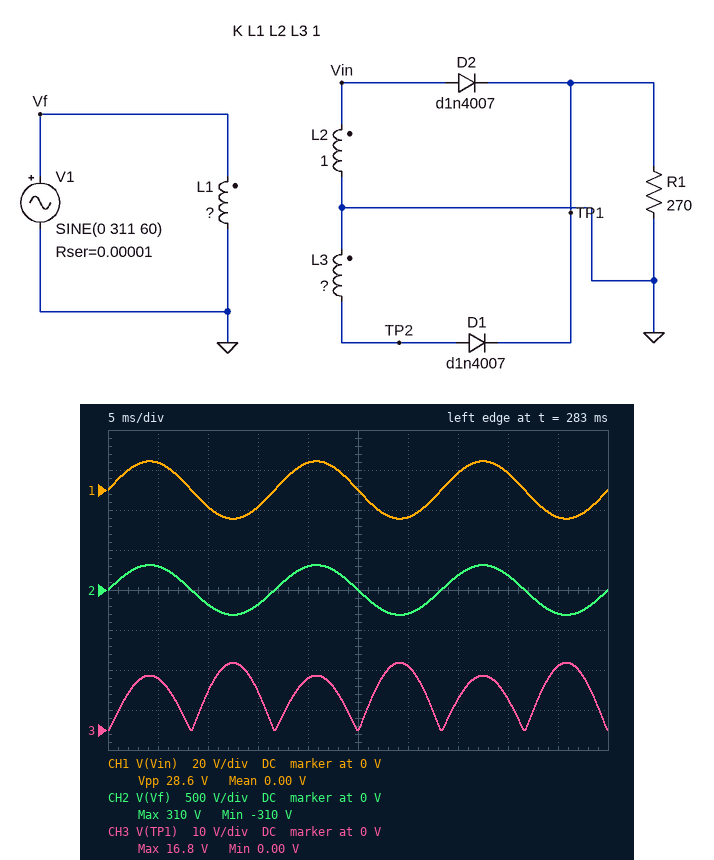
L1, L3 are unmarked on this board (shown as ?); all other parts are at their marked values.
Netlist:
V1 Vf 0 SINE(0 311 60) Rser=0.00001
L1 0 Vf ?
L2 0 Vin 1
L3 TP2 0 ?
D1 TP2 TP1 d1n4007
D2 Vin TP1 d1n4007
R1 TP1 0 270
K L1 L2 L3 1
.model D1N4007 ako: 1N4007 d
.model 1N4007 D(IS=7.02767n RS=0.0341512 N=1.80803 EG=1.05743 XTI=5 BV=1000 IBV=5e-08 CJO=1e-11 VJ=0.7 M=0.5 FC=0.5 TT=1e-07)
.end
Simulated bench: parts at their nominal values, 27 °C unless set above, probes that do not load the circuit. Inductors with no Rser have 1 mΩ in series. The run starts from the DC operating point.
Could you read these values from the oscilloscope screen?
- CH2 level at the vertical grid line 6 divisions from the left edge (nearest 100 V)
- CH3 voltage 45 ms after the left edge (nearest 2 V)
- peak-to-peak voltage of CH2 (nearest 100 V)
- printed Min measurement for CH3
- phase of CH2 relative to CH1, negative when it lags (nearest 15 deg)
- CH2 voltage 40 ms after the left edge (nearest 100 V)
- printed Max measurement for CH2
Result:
-300 V
16 V
600 V
0.00 V
0 deg
200 V
310 V
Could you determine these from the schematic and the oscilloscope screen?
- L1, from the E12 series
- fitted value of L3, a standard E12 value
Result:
470 H
1.5 H
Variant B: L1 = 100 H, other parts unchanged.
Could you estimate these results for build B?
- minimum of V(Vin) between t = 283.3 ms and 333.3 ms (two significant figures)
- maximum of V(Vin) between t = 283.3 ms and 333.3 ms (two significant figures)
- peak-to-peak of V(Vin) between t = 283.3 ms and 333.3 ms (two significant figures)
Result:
-31 V
31 V
62 V
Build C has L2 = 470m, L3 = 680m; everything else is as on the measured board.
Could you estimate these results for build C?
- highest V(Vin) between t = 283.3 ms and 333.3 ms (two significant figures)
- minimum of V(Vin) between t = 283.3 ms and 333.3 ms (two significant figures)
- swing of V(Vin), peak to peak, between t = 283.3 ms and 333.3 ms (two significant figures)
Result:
9.8 V
-9.8 V
20 V
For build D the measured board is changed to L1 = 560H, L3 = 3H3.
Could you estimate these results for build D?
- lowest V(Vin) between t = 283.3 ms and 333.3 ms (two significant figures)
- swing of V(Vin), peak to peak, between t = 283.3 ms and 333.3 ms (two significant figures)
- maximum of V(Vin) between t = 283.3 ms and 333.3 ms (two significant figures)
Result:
-13 V
26 V
13 V
